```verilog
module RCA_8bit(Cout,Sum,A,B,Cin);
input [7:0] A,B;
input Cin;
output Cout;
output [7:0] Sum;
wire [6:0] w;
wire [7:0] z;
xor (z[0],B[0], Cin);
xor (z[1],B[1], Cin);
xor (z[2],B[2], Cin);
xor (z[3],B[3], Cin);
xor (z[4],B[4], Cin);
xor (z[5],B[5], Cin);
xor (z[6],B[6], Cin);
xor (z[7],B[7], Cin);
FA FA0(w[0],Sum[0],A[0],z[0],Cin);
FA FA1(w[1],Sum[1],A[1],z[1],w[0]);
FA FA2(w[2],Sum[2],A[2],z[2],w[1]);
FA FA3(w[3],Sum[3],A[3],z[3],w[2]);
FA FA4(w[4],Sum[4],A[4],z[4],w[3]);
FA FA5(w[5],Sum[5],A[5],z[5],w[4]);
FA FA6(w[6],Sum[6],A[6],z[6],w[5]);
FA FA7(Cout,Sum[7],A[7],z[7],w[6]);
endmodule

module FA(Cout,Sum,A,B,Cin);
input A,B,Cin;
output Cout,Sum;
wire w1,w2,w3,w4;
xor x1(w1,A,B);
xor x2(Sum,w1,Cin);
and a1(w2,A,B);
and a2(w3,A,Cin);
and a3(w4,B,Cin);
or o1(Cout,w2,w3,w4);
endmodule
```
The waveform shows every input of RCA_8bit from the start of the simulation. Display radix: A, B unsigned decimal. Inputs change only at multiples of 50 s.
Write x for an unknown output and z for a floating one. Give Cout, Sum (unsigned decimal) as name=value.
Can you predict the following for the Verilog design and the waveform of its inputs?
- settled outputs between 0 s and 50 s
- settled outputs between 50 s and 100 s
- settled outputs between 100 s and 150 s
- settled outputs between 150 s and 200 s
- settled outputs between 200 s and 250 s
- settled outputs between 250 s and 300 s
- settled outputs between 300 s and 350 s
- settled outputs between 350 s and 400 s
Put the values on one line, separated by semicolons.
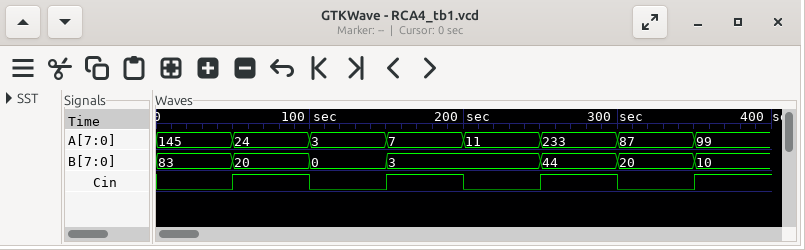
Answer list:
Cout=0, Sum=228; Cout=1, Sum=4; Cout=0, Sum=3; Cout=1, Sum=4; Cout=0, Sum=14; Cout=1, Sum=189; Cout=0, Sum=107; Cout=1, Sum=89
